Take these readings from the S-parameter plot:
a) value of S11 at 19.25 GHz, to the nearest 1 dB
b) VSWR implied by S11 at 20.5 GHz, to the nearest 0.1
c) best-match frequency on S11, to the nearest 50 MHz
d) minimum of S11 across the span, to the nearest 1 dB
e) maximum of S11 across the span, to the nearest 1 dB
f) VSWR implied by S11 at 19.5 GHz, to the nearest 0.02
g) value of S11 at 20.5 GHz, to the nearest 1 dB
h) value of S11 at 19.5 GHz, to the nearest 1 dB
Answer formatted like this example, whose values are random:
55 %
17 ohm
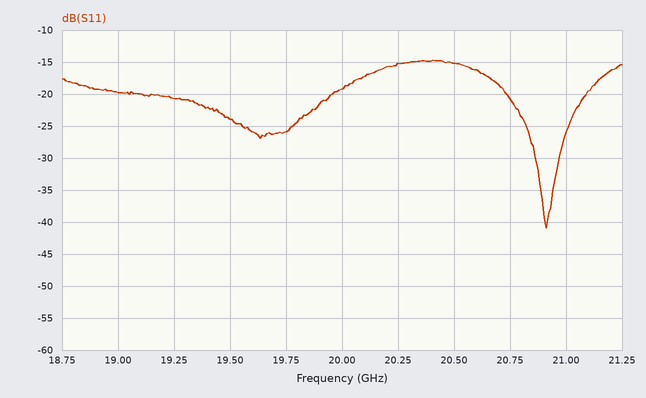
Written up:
-21 dB
1.4
20.90 GHz
-41 dB
-15 dB
1.14
-15 dB
-24 dB
